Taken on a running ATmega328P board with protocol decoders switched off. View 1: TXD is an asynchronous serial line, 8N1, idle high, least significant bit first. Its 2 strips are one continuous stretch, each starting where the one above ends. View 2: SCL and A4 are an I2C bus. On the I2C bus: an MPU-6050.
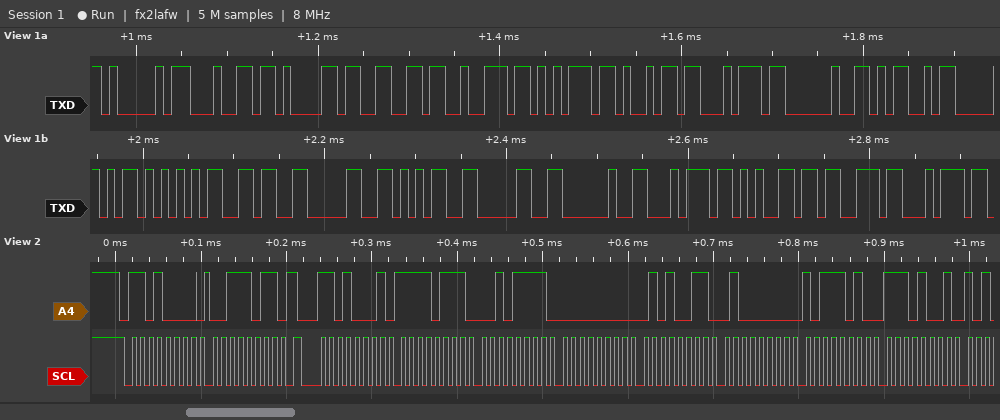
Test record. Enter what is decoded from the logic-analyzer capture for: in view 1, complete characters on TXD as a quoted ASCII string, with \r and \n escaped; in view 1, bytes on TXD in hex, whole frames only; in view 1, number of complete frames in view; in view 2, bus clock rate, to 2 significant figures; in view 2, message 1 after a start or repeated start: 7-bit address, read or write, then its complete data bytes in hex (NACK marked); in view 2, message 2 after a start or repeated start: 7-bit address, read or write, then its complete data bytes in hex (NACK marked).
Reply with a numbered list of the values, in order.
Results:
1. "Adafruit MPU6050 test"
2. 41 64 61 66 72 75 69 74 20 4D 50 55 36 30 35 30 20 74 65 73 74
3. 21
4. 100 kHz
5. 0x68 write: 3B
6. 0x68 read: F7 2F 00 53 40 BA E9
